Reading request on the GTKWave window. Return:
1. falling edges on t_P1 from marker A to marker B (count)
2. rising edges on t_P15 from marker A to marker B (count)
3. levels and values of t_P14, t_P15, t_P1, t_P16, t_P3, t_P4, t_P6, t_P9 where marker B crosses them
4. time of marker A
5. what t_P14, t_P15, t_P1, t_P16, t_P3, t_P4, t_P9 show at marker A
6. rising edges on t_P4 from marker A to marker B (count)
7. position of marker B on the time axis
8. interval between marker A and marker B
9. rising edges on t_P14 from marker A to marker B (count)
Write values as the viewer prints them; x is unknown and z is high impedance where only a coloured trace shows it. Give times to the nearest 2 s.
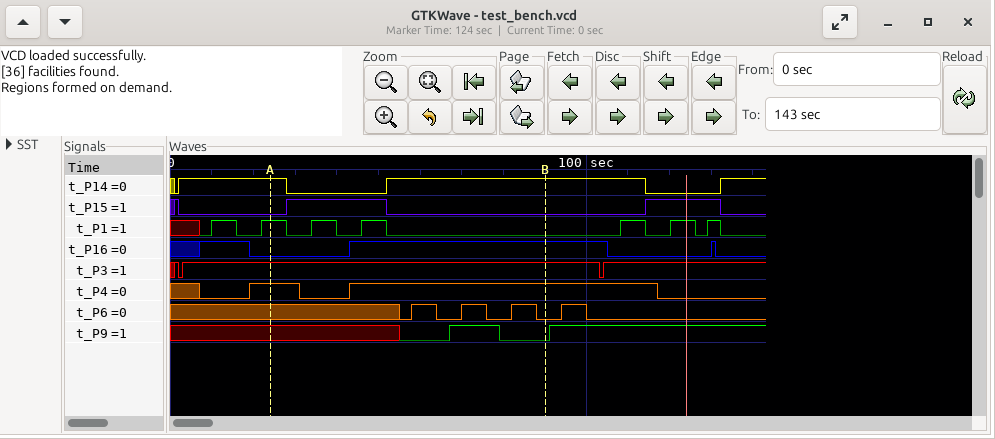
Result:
3
1
t_P14=1, t_P15=0, t_P1=0, t_P16=1, t_P3=1, t_P4=1, t_P6=0, t_P9=0
24 s
t_P14=1, t_P15=0, t_P1=1, t_P16=0, t_P3=1, t_P4=1, t_P9=x
1
90 s
66 s
1
